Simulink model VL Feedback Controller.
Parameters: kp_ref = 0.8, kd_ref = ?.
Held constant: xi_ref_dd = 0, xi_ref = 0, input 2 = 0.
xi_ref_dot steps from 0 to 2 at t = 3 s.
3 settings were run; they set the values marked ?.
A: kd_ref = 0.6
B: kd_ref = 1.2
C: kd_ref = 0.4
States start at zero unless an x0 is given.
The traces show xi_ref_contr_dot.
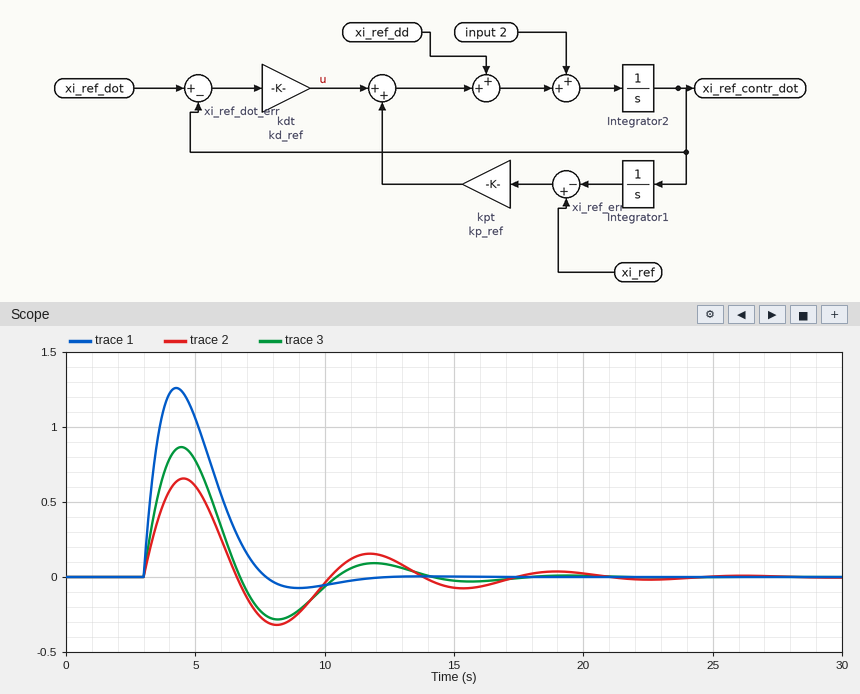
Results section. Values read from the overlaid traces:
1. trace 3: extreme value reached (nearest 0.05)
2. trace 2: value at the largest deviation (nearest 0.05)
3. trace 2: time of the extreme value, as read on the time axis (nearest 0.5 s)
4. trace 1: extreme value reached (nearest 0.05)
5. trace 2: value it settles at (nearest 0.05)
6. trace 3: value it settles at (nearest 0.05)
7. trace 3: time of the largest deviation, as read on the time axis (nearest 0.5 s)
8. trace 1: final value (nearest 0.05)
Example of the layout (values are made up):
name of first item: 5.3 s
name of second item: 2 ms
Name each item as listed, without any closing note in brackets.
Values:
trace 3: extreme value reached: 0.85
trace 2: value at the largest deviation: 0.65
trace 2: time of the extreme value, as read on the time axis: 4.5 s
trace 1: extreme value reached: 1.25
trace 2: value it settles at: 0.00
trace 3: value it settles at: 0.00
trace 3: time of the largest deviation, as read on the time axis: 4.5 s
trace 1: final value: 0.00
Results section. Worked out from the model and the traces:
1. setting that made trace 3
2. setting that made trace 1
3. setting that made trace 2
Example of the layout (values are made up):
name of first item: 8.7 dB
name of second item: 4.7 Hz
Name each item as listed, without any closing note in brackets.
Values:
setting that made trace 3: A
setting that made trace 1: B
setting that made trace 2: C
